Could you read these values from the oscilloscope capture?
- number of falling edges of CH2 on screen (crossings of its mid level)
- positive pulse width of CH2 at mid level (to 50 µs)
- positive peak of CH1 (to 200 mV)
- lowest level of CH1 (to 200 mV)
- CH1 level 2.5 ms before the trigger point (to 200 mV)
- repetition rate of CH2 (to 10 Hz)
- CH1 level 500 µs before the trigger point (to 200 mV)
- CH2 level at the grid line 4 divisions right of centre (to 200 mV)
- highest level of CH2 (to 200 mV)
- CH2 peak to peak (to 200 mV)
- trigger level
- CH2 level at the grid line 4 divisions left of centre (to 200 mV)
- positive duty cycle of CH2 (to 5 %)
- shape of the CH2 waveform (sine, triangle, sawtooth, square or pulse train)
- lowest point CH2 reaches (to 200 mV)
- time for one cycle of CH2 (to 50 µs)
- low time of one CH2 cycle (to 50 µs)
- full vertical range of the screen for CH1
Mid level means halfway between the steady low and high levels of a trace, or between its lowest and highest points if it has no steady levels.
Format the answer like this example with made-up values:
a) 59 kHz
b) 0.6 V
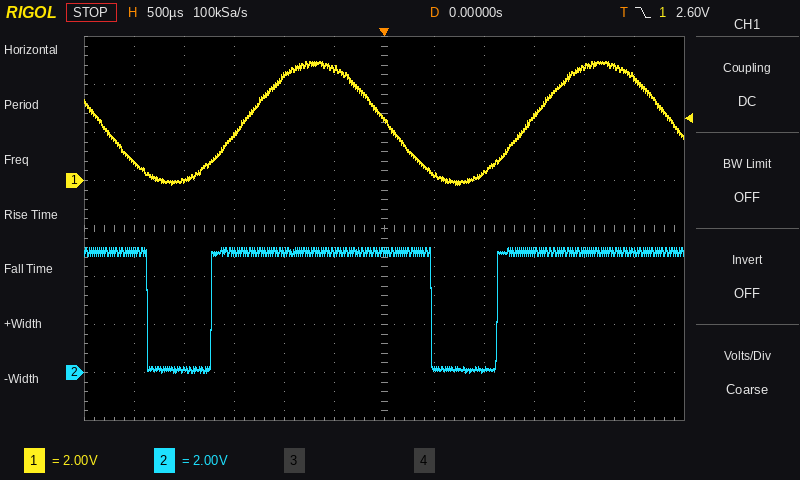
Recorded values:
a) 2
b) 2.20 ms
c) 5.0 V
d) -200 mV
e) 800 mV
f) 350 Hz
g) 4.6 V
h) 5.0 V
i) 5.2 V
j) 5.2 V
k) 2.60 V
l) 200 mV
m) 75 %
n) pulse train
o) 0.0 V
p) 2.85 ms
q) 650 µs
r) 16 V
